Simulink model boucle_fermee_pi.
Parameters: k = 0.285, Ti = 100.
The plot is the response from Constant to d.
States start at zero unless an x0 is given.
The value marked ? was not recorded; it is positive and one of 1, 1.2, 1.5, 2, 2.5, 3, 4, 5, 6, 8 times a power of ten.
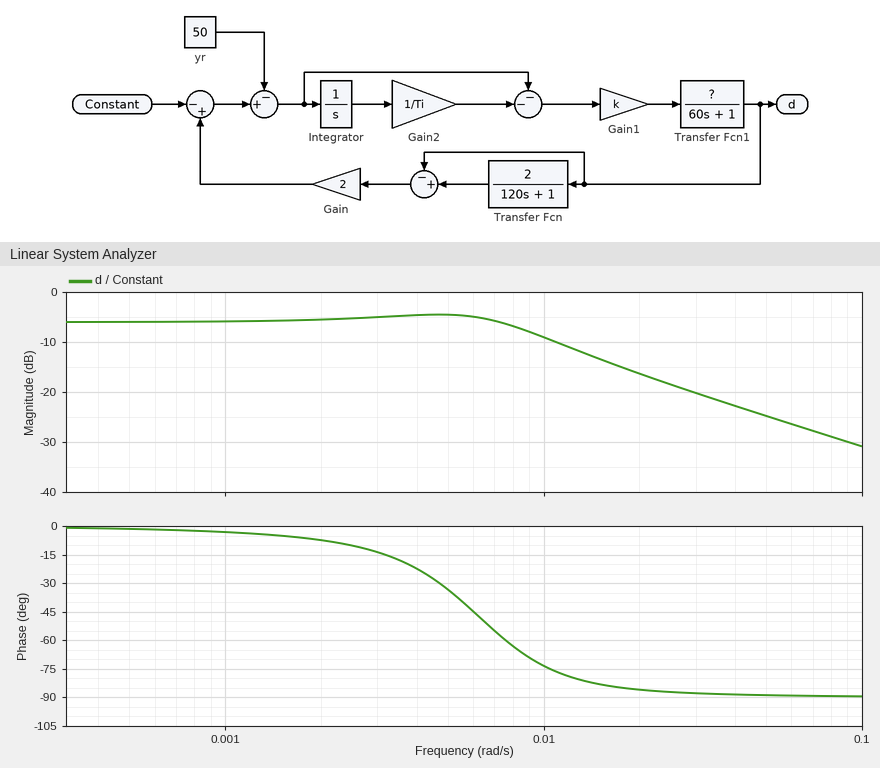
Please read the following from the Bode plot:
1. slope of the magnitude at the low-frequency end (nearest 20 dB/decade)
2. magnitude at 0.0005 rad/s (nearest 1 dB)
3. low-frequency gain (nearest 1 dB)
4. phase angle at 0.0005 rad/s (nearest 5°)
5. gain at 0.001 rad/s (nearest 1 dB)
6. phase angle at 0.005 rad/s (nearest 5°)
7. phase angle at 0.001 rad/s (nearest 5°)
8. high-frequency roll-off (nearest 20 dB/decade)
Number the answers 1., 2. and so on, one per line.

1. 0 dB/decade
2. -6 dB
3. -6 dB
4. 0°
5. -6 dB
6. -35°
7. -5°
8. -20 dB/decade
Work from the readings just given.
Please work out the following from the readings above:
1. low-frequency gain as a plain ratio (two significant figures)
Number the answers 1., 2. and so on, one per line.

1. 0.50
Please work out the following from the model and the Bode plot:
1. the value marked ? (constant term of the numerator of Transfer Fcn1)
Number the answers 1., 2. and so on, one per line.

1. 0.6
